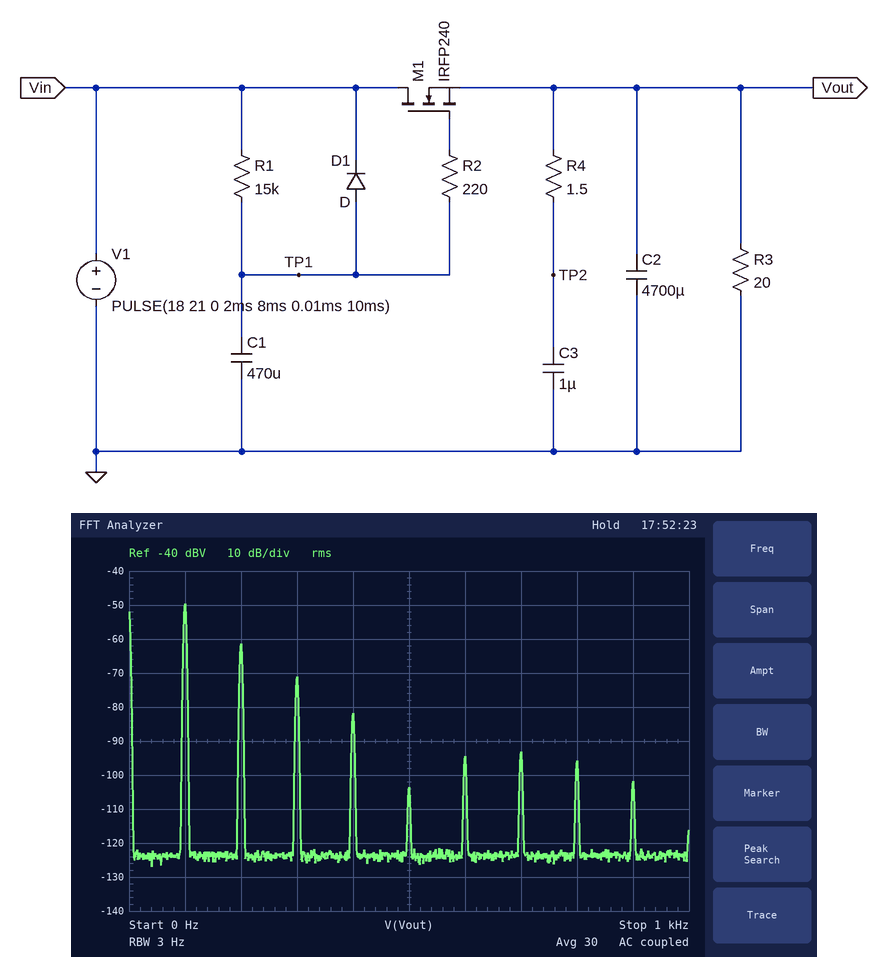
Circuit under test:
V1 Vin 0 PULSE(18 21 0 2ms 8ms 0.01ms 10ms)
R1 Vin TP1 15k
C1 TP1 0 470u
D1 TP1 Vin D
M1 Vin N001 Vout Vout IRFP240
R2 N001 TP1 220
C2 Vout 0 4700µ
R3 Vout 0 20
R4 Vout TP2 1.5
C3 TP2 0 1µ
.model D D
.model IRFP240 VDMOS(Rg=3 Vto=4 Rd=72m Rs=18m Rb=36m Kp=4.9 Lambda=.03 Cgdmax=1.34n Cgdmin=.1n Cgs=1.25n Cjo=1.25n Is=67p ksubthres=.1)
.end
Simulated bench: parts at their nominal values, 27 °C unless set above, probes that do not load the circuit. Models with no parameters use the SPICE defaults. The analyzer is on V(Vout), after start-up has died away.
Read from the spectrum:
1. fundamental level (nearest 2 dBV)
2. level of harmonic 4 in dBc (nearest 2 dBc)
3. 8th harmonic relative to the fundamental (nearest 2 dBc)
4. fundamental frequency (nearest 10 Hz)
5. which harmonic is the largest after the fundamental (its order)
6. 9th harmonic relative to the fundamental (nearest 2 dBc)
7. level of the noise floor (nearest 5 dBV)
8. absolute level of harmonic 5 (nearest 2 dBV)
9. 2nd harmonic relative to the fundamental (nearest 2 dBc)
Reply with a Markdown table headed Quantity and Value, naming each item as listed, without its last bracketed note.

| Quantity | Value |
|---|---|
| fundamental level | -50 dBV |
| level of harmonic 4 in dBc | -32 dBc |
| 8th harmonic relative to the fundamental | -46 dBc |
| fundamental frequency | 100 Hz |
| which harmonic is the largest after the fundamental | 2 |
| 9th harmonic relative to the fundamental | -52 dBc |
| level of the noise floor | -125 dBV |
| absolute level of harmonic 5 | -104 dBV |
| 2nd harmonic relative to the fundamental | -12 dBc |
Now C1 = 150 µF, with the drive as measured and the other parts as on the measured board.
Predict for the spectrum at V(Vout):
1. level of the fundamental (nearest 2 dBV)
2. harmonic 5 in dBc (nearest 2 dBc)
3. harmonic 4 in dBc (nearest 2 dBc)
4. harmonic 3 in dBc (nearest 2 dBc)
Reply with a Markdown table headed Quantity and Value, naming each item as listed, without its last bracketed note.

| Quantity | Value |
|---|---|
| level of the fundamental | -50 dBV |
| harmonic 5 in dBc | -42 dBc |
| harmonic 4 in dBc | -30 dBc |
| harmonic 3 in dBc | -20 dBc |
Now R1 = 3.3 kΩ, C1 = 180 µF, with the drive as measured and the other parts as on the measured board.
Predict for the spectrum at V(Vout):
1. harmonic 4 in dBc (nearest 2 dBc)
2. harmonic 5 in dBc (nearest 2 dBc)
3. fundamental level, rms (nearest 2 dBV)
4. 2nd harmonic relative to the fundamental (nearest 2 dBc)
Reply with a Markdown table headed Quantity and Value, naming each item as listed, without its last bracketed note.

| Quantity | Value |
|---|---|
| harmonic 4 in dBc | -24 dBc |
| harmonic 5 in dBc | -30 dBc |
| fundamental level, rms | -50 dBV |
| 2nd harmonic relative to the fundamental | -10 dBc |
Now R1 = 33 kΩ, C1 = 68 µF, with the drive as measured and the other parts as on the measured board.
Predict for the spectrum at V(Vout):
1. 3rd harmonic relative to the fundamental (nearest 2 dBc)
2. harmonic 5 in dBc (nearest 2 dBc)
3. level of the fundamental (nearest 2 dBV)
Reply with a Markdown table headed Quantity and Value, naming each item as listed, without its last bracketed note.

| Quantity | Value |
|---|---|
| 3rd harmonic relative to the fundamental | -20 dBc |
| harmonic 5 in dBc | -42 dBc |
| level of the fundamental | -50 dBV |
